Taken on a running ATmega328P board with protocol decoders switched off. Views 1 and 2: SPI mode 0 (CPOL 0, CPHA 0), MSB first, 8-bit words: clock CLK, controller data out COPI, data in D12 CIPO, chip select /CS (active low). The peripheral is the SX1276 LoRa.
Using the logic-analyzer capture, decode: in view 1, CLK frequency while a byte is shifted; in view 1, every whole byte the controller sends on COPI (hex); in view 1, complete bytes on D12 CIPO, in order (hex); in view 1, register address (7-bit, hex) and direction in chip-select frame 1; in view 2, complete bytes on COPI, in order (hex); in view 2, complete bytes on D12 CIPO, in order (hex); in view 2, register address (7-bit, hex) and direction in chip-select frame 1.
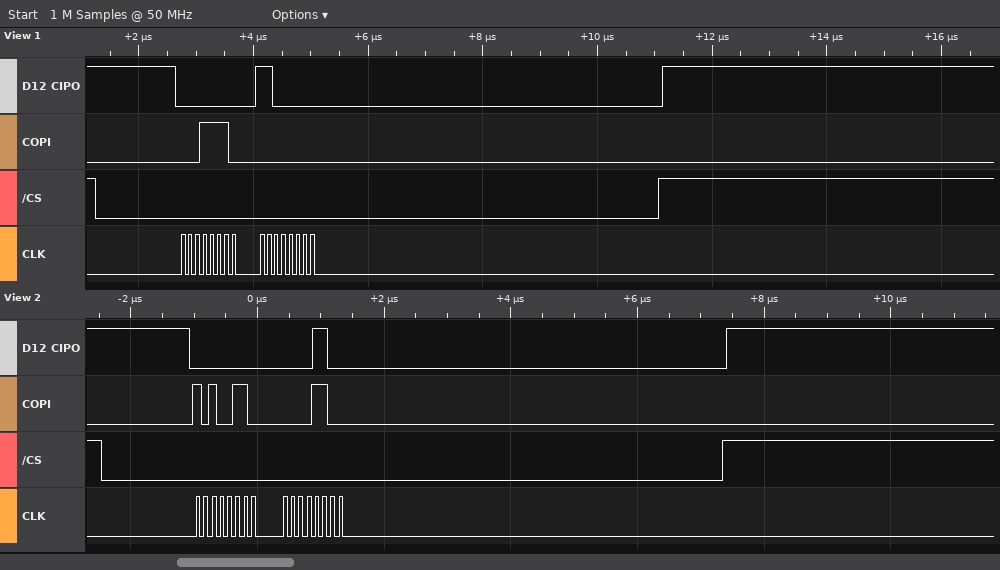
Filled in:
8 MHz
1E 00
00 C0
0x1E read
A6 0C
00 0C
0x26 write
